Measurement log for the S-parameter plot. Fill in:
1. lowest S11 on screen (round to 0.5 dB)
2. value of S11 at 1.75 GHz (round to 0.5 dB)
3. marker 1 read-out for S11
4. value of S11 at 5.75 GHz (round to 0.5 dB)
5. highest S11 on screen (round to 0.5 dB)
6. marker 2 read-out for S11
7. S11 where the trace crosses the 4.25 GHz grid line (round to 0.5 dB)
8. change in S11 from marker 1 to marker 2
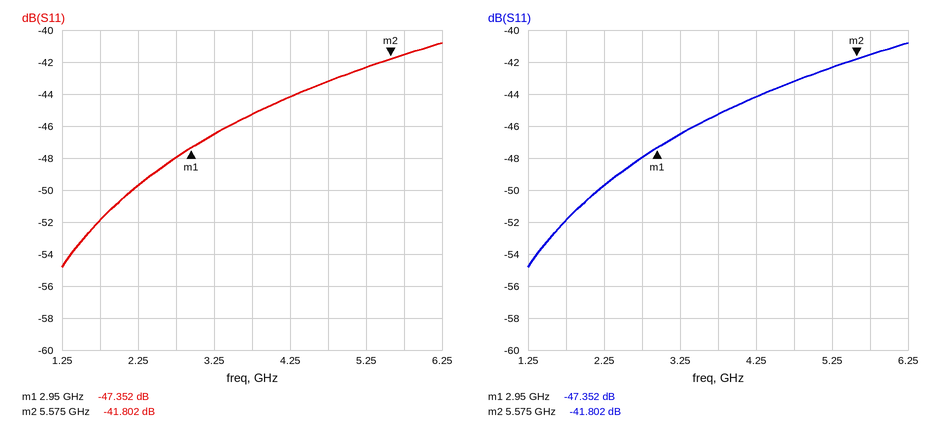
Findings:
-55.0 dB
-52.0 dB
-47.352 dB
-41.5 dB
-41.0 dB
-41.802 dB
-44.0 dB
5.550 dB
